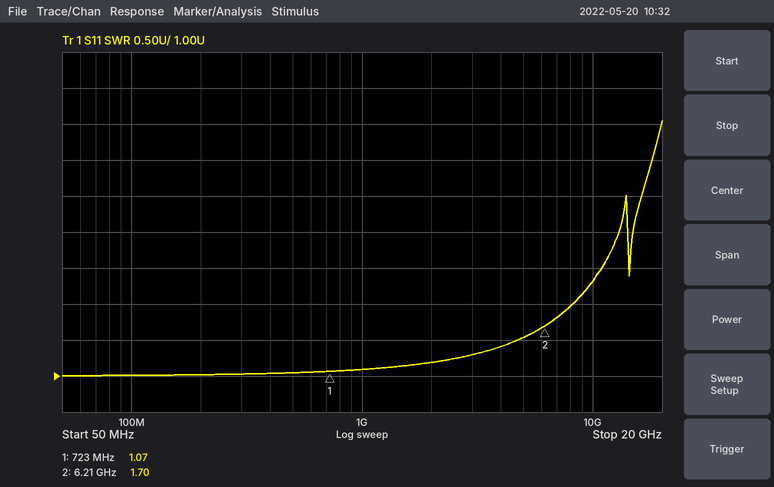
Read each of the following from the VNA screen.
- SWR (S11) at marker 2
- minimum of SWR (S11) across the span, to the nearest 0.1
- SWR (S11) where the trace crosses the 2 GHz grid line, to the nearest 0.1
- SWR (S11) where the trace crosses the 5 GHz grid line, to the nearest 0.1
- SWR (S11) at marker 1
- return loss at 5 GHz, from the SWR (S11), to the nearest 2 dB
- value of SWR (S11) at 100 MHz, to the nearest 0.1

1.70
1.0
1.2
1.5
1.07
14 dB
1.0
